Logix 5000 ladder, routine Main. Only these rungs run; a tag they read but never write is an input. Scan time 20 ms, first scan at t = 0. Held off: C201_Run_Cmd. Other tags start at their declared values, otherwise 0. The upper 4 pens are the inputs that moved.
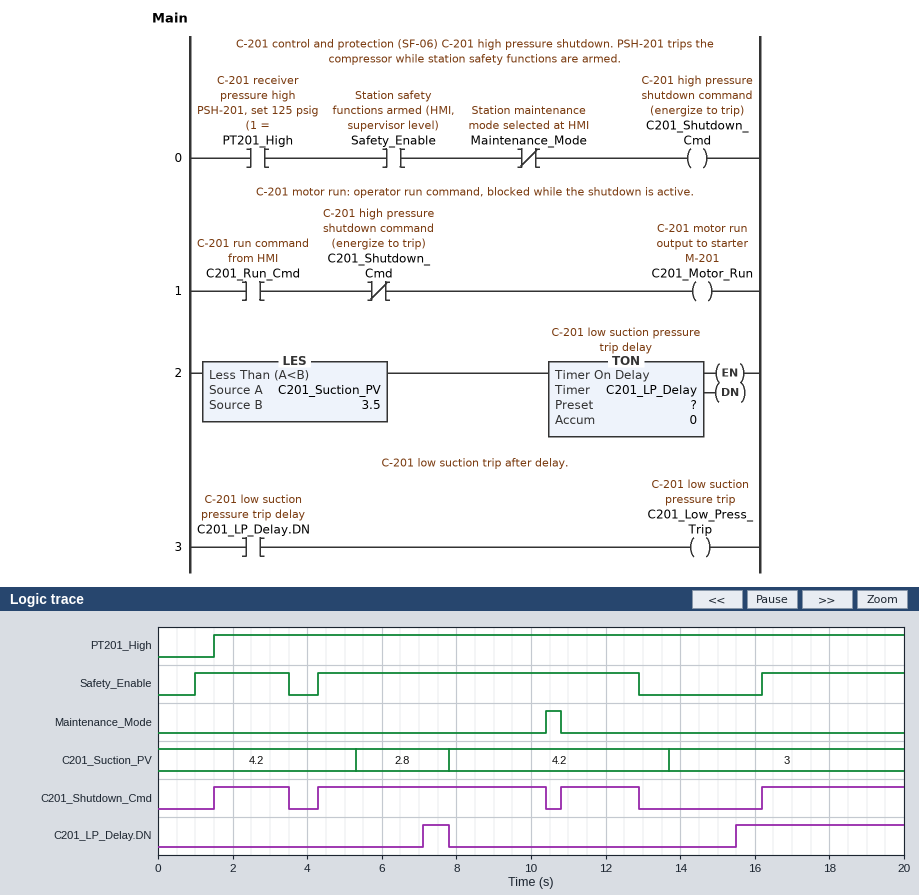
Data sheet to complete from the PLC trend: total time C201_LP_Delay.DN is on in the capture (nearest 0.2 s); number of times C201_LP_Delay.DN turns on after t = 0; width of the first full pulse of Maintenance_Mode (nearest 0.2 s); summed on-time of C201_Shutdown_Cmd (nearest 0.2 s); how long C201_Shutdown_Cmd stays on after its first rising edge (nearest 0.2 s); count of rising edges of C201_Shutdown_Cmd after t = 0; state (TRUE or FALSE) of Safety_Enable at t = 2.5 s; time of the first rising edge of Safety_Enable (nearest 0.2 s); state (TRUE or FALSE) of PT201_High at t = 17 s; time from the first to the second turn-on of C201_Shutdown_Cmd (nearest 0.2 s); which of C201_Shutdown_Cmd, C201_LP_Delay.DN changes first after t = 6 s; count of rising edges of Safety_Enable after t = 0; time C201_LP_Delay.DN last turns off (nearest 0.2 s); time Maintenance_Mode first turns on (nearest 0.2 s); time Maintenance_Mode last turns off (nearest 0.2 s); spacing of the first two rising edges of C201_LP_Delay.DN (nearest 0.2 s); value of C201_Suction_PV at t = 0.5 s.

5.2 s
2
0.4 s
14.0 s
2.0 s
4
TRUE
1.0 s
TRUE
2.8 s
C201_LP_Delay.DN
3
7.8 s
10.4 s
10.8 s
8.4 s
4.2
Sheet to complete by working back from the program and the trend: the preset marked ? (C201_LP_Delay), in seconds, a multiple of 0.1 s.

1.8 s
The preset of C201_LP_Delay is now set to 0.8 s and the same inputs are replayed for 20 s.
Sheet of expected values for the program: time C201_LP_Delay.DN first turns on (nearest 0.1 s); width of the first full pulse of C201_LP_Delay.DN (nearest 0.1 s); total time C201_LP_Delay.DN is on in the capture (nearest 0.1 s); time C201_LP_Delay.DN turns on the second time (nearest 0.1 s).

6.1 s
1.7 s
7.2 s
14.5 s
